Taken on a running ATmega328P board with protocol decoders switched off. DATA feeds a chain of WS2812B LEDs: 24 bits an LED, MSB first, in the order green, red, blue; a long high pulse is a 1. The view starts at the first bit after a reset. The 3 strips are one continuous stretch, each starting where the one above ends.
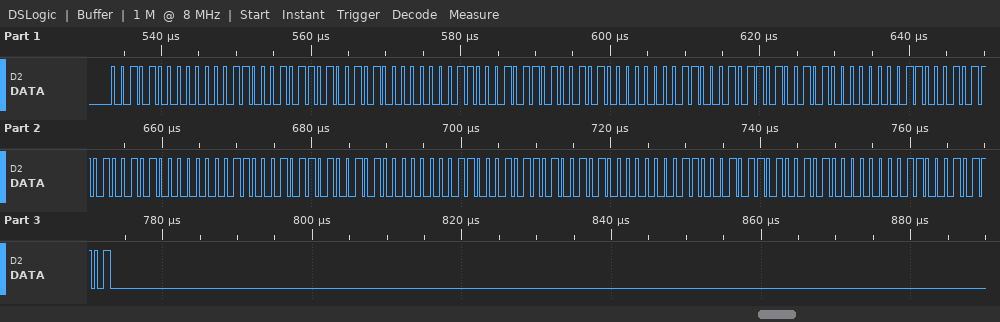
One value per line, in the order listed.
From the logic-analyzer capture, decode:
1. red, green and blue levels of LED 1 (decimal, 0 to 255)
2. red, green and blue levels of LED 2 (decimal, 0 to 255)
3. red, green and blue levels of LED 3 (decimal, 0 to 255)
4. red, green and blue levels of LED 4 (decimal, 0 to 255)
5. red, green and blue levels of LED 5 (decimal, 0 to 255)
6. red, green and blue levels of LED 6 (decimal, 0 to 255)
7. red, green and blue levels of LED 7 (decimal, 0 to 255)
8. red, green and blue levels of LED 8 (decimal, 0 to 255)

6, 40, 45
6, 40, 45
6, 40, 45
6, 40, 45
6, 40, 45
6, 40, 45
6, 40, 45
6, 40, 45
